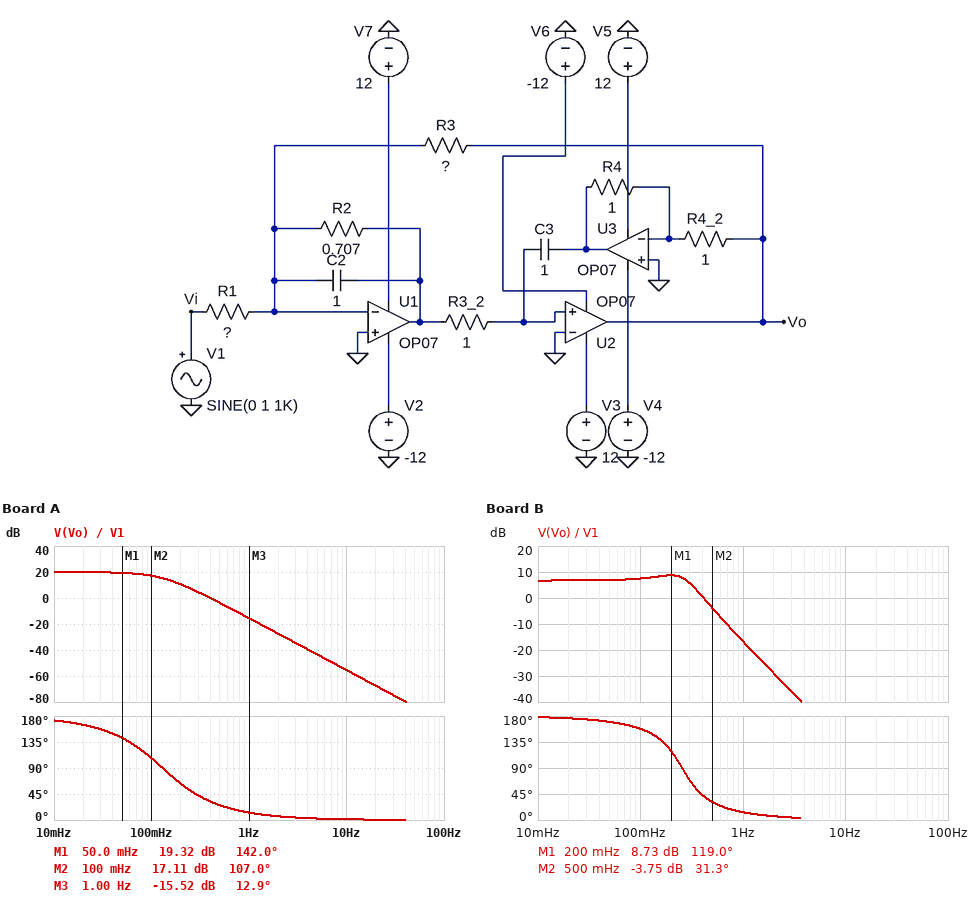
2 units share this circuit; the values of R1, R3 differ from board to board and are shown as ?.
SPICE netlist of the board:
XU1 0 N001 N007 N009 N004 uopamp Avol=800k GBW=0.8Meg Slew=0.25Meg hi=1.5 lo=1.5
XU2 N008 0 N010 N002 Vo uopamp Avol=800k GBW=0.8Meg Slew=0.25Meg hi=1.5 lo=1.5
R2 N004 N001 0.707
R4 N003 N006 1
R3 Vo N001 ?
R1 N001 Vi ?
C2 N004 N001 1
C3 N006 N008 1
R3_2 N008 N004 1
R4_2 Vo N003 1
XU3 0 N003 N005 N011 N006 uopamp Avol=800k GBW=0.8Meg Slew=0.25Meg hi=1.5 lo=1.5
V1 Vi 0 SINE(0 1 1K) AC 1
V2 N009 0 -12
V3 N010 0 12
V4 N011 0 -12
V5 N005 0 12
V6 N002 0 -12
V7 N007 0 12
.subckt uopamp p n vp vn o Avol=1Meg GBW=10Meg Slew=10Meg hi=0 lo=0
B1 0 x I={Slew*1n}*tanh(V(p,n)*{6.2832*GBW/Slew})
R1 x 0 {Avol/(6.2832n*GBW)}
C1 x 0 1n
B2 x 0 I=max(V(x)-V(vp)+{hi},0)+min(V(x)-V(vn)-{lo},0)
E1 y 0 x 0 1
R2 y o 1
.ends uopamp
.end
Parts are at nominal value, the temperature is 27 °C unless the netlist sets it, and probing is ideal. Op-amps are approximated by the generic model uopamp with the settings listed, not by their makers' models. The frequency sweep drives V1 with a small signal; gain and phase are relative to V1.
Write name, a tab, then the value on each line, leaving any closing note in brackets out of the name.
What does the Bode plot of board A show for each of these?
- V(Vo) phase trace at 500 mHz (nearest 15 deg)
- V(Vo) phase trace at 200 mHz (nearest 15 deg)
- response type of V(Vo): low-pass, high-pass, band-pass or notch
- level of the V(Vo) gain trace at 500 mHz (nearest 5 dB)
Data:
V(Vo) phase trace at 500 mHz	30 deg
V(Vo) phase trace at 200 mHz	60 deg
response type of V(Vo): low-pass, high-pass, band-pass or notch	low-pass
level of the V(Vo) gain trace at 500 mHz	-5 dB
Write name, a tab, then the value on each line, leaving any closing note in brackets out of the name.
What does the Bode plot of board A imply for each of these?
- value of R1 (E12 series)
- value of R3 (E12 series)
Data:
value of R1	0.15 Ω
value of R3	1.5 Ω
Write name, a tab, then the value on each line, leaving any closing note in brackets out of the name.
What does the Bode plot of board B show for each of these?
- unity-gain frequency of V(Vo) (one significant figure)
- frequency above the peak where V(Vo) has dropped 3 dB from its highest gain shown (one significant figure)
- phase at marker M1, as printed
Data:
unity-gain frequency of V(Vo)	400 mHz
frequency above the peak where V(Vo) has dropped 3 dB from its highest gain shown	300 mHz
phase at marker M1, as printed	119.0 deg
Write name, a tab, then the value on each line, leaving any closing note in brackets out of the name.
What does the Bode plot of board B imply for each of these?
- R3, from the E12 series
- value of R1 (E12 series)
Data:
R3, from the E12 series	0.39 Ω
value of R1	0.18 Ω
